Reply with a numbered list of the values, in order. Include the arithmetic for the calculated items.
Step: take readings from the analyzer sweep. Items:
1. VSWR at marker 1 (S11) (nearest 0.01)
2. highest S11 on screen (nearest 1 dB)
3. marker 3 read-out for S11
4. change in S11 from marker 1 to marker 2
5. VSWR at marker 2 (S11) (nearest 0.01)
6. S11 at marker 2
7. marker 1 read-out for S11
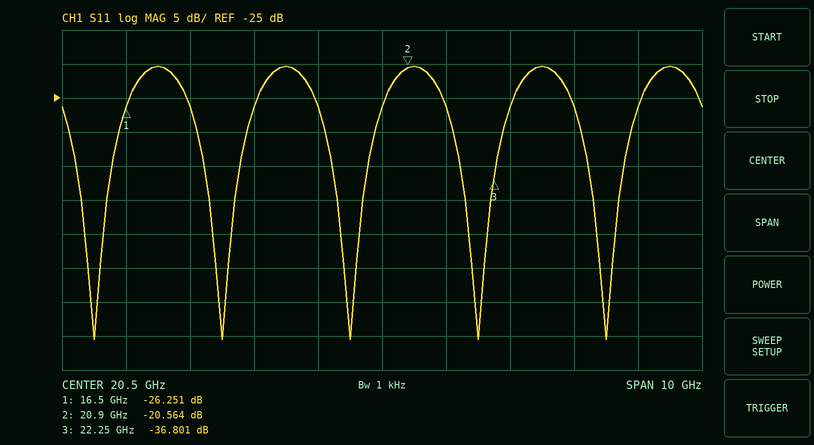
1. (1 + 0.0487)/(1 − 0.0487) ≈ 1.10
2. -20 dB
3. -36.801 dB
4. -20.564 − (-26.251) = 5.687 dB
5. (1 + 0.0937)/(1 − 0.0937) ≈ 1.21
6. -20.564 dB
7. -26.251 dB
